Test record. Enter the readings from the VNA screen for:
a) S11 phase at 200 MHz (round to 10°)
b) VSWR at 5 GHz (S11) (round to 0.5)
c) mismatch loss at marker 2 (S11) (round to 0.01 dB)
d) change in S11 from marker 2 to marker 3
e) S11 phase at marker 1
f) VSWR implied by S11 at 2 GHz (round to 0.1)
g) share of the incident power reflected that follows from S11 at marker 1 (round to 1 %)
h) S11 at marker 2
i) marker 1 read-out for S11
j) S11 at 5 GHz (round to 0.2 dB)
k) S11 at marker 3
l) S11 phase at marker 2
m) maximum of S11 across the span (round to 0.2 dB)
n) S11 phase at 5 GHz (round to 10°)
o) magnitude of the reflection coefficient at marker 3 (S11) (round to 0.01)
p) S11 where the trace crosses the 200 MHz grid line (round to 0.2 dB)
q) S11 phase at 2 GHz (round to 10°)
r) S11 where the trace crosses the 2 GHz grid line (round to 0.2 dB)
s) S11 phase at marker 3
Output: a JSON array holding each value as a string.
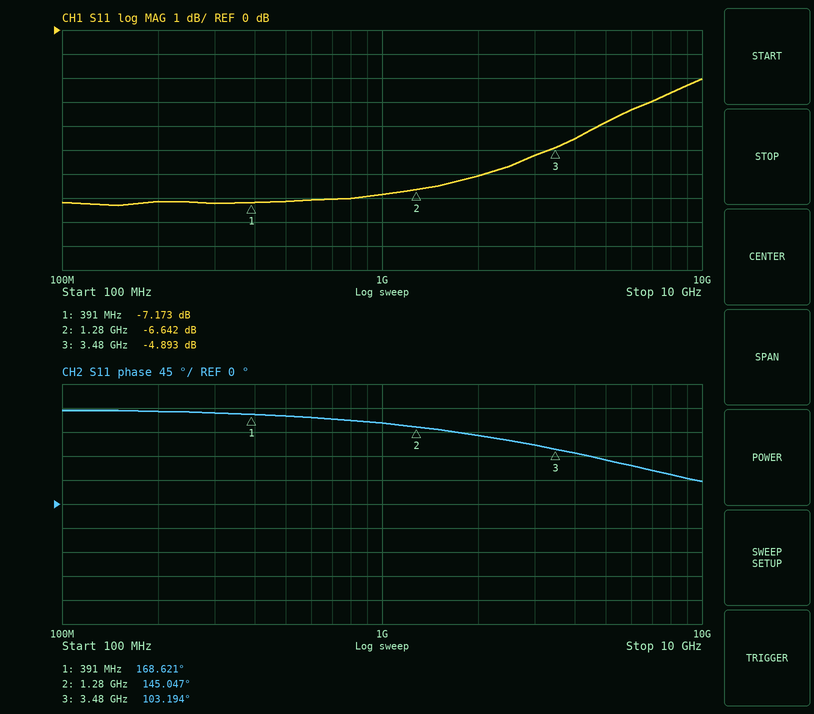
["170°", "4.5", "1.06 dB", "1.749 dB", "168.621°", "3.0", "19 %", "-6.642 dB", "-7.173 dB", "-3.8 dB", "-4.893 dB", "145.047°", "-2.0 dB", "80°", "0.57", "-7.2 dB", "130°", "-6.0 dB", "103.194°"]
